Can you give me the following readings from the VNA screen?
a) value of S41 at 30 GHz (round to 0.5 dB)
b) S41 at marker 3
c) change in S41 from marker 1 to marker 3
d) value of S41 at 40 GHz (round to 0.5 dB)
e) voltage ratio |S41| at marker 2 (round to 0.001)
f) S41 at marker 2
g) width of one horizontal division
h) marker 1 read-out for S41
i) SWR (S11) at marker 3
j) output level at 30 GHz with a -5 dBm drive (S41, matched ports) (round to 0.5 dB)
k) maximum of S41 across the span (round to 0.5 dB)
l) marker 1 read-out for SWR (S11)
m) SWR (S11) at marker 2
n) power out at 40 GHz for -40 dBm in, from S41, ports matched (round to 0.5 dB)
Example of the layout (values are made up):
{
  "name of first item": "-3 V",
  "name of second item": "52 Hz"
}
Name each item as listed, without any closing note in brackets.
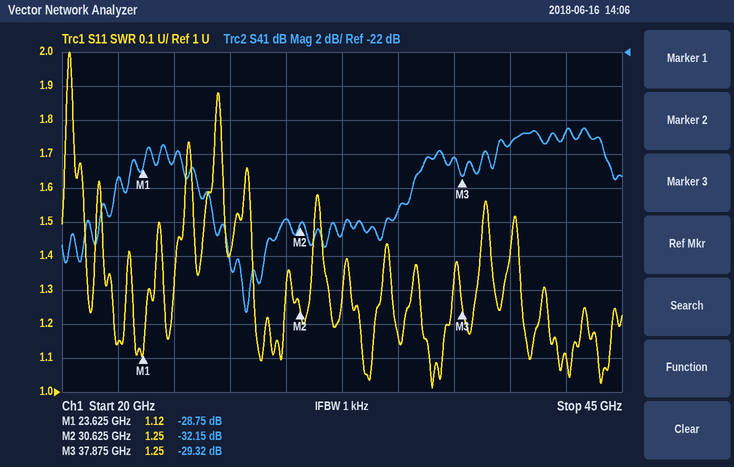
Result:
{
  "value of S41 at 30 GHz": "-32.0 dB",
  "S41 at marker 3": "-29.32 dB",
  "change in S41 from marker 1 to marker 3": "-0.57 dB",
  "value of S41 at 40 GHz": "-27.5 dB",
  "voltage ratio |S41| at marker 2": "0.025",
  "S41 at marker 2": "-32.15 dB",
  "width of one horizontal division": "2.5 GHz",
  "marker 1 read-out for S41": "-28.75 dB",
  "SWR (S11) at marker 3": "1.25",
  "output level at 30 GHz with a -5 dBm drive (S41, matched ports)": "-37.0 dBm",
  "maximum of S41 across the span": "-26.5 dB",
  "marker 1 read-out for SWR": "1.12",
  "SWR (S11) at marker 2": "1.25",
  "power out at 40 GHz for -40 dBm in, from S41, ports matched": "-67.5 dBm"
}
